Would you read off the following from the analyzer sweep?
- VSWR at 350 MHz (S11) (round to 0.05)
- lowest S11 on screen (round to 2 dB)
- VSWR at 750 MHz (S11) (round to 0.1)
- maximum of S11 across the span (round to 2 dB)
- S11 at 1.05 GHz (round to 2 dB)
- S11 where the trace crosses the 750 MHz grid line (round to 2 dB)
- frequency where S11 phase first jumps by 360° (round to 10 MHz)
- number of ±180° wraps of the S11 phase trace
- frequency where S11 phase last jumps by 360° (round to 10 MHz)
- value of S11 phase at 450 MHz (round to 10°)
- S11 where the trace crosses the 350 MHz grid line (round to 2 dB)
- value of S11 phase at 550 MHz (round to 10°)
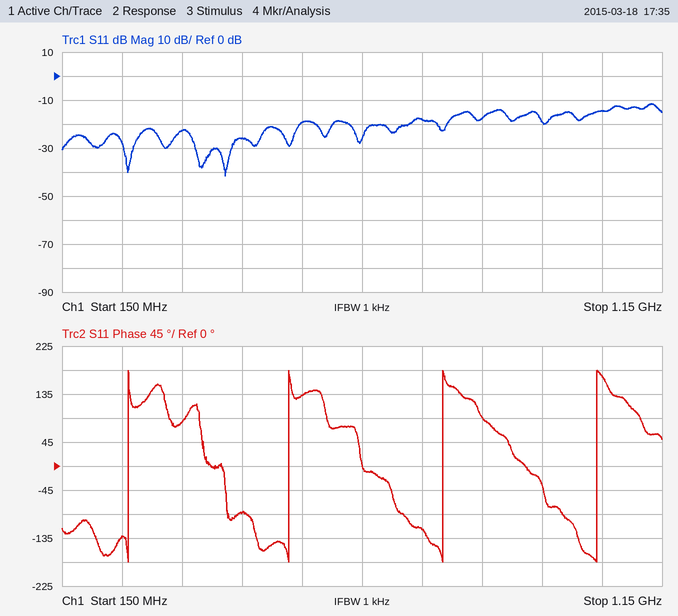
1.15
-42 dB
1.3
-12 dB
-14 dB
-18 dB
260 MHz
4
1.04 GHz
-90°
-22 dB
130°
